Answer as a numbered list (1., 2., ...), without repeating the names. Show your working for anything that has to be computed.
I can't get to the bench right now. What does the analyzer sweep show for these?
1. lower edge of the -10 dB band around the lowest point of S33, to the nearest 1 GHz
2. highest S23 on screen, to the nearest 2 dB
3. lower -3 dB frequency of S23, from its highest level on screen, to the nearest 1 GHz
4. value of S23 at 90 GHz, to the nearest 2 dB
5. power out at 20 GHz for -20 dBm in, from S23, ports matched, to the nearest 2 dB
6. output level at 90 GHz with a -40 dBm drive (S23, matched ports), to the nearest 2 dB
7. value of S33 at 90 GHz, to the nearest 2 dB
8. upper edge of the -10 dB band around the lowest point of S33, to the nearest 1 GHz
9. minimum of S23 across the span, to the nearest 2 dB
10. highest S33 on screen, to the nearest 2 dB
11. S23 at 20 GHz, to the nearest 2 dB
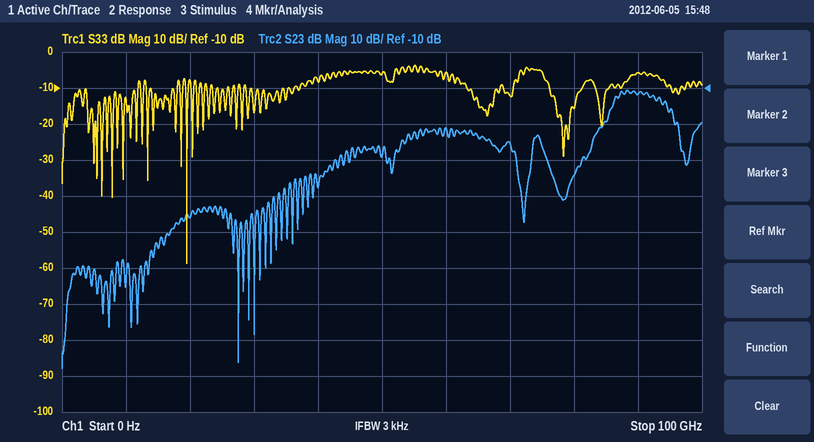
1. 19 GHz
2. -10 dB
3. 86 GHz
4. -12 dB
5. -20 dBm + (-46 dB) = -66 dBm
6. -40 dBm + (-12 dB) = -52 dBm
7. -6 dB
8. 20 GHz
9. -88 dB
10. -4 dB
11. -46 dB
